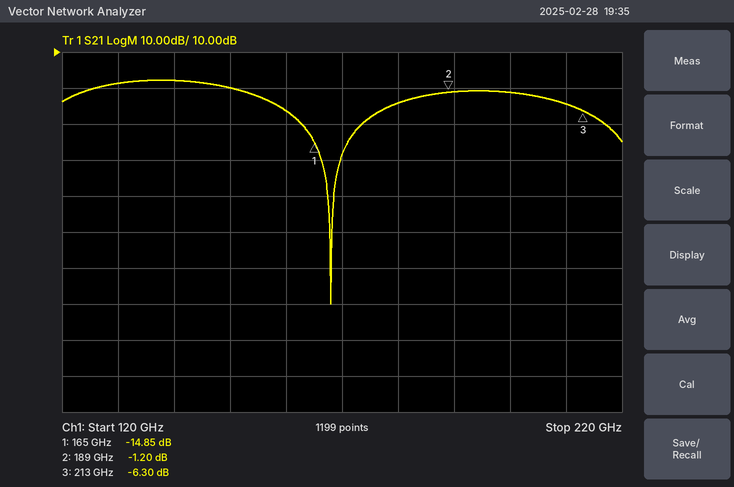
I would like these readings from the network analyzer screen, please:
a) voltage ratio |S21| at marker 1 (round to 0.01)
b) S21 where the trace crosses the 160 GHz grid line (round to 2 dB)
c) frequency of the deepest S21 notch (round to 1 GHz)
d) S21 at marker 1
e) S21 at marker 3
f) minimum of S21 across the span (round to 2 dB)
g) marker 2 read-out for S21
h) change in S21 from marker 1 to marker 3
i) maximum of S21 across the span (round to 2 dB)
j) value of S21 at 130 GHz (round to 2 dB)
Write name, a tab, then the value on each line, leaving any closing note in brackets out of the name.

voltage ratio |S21| at marker 1	0.18
S21 where the trace crosses the 160 GHz grid line	-6 dB
frequency of the deepest S21 notch	168 GHz
S21 at marker 1	-14.85 dB
S21 at marker 3	-6.30 dB
minimum of S21 across the span	-60 dB
marker 2 read-out for S21	-1.20 dB
change in S21 from marker 1 to marker 3	8.55 dB
maximum of S21 across the span	2 dB
value of S21 at 130 GHz	2 dB
